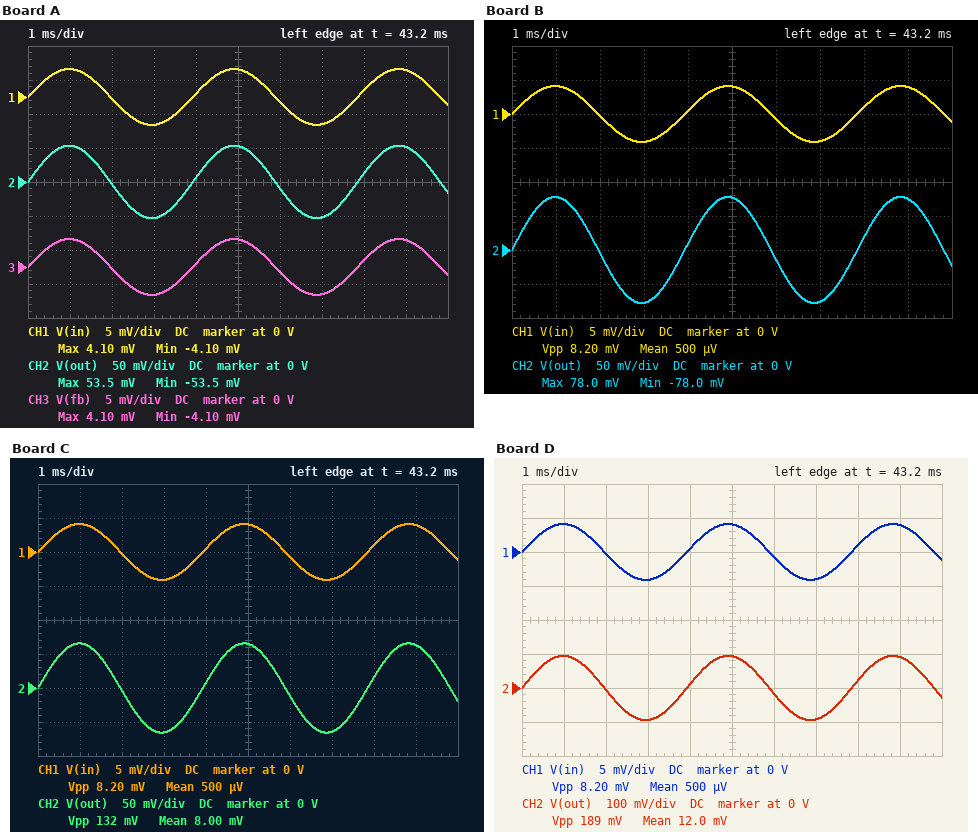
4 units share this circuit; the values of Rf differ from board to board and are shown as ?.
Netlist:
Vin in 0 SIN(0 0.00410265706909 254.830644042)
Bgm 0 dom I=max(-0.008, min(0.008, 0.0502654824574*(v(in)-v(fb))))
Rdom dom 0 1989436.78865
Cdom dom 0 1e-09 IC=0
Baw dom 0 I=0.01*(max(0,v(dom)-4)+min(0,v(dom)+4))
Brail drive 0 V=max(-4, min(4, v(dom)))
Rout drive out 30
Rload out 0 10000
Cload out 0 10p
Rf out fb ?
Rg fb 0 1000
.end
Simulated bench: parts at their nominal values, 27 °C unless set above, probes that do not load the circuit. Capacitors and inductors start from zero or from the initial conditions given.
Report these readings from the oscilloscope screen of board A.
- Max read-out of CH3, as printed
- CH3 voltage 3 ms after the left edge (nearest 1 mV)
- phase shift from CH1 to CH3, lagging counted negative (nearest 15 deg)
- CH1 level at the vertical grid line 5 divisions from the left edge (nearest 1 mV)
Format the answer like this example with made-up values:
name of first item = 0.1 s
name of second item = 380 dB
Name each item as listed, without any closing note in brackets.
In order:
Max read-out of CH3, as printed = 4.10 mV
CH3 voltage 3 ms after the left edge = -4 mV
phase shift from CH1 to CH3, lagging counted negative = 0 deg
CH1 level at the vertical grid line 5 divisions from the left edge = 4 mV
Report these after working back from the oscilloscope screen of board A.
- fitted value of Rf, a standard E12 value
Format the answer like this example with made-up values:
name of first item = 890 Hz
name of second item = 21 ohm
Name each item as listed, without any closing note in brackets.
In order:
fitted value of Rf, a standard E12 value = 12 kΩ
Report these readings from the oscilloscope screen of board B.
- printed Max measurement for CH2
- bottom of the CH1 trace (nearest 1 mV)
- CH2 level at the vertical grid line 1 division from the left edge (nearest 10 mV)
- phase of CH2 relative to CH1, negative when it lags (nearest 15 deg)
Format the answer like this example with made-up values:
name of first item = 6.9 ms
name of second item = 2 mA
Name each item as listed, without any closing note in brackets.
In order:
printed Max measurement for CH2 = 78.0 mV
bottom of the CH1 trace = -4 mV
CH2 level at the vertical grid line 1 division from the left edge = 80 mV
phase of CH2 relative to CH1, negative when it lags = 0 deg
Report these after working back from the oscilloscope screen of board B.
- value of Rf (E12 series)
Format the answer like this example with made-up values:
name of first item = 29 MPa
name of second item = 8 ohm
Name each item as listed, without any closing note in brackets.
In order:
value of Rf = 18 kΩ
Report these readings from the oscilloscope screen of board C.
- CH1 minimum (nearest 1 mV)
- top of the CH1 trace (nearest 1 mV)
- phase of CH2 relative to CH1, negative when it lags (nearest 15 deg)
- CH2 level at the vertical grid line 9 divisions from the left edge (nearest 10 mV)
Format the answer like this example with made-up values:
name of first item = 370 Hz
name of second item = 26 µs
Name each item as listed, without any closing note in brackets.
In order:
CH1 minimum = -4 mV
top of the CH1 trace = 4 mV
phase of CH2 relative to CH1, negative when it lags = 0 deg
CH2 level at the vertical grid line 9 divisions from the left edge = 60 mV
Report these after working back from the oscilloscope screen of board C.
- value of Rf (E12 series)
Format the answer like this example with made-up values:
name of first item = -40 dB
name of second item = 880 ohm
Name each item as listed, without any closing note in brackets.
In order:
value of Rf = 15 kΩ
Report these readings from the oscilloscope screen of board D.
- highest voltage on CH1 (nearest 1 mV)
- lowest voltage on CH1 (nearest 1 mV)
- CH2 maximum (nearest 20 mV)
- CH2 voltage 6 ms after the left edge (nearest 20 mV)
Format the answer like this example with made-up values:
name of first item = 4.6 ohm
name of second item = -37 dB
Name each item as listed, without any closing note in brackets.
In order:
highest voltage on CH1 = 4 mV
lowest voltage on CH1 = -4 mV
CH2 maximum = 100 mV
CH2 voltage 6 ms after the left edge = -20 mV
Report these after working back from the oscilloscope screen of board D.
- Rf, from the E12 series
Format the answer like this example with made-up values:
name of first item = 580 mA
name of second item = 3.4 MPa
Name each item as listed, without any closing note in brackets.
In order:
Rf, from the E12 series = 22 kΩ
